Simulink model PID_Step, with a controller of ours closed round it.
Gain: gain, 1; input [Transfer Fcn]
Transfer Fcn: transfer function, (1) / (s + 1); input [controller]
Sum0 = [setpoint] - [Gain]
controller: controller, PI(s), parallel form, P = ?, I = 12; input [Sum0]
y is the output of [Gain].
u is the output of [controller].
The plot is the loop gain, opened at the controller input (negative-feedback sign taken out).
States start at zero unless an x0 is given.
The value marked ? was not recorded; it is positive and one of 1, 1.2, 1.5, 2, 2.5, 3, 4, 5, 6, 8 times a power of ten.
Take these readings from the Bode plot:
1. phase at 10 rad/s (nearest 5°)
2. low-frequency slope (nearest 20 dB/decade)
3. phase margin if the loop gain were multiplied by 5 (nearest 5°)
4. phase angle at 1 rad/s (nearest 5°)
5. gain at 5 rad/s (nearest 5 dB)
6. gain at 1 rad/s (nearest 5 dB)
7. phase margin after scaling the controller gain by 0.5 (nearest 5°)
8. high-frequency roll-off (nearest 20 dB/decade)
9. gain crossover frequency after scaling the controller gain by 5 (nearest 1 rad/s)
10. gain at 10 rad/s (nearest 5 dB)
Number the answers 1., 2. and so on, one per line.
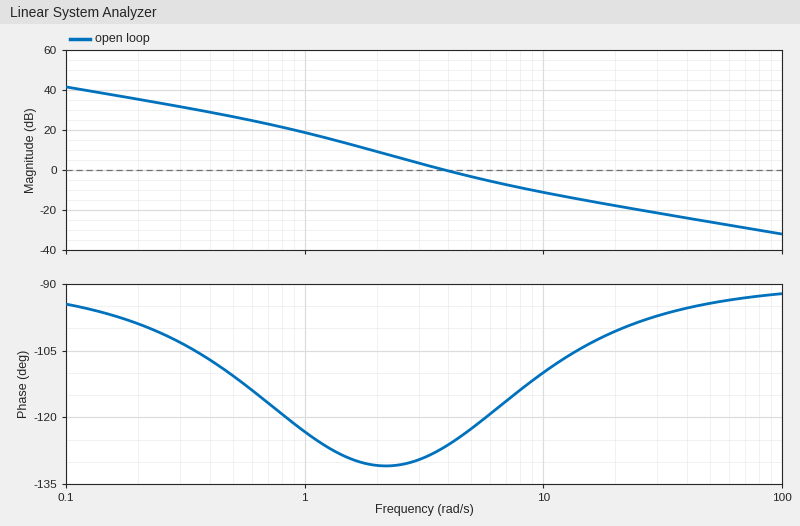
1. -110°
2. -20 dB/decade
3. 75°
4. -125°
5. -5 dB
6. 20 dB
7. 50°
8. -20 dB/decade
9. 13 rad/s
10. -10 dB
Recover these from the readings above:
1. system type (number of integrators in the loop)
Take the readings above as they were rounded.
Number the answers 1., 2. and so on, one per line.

1. 1
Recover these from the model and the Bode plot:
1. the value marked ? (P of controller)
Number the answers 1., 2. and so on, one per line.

1. 2.5
